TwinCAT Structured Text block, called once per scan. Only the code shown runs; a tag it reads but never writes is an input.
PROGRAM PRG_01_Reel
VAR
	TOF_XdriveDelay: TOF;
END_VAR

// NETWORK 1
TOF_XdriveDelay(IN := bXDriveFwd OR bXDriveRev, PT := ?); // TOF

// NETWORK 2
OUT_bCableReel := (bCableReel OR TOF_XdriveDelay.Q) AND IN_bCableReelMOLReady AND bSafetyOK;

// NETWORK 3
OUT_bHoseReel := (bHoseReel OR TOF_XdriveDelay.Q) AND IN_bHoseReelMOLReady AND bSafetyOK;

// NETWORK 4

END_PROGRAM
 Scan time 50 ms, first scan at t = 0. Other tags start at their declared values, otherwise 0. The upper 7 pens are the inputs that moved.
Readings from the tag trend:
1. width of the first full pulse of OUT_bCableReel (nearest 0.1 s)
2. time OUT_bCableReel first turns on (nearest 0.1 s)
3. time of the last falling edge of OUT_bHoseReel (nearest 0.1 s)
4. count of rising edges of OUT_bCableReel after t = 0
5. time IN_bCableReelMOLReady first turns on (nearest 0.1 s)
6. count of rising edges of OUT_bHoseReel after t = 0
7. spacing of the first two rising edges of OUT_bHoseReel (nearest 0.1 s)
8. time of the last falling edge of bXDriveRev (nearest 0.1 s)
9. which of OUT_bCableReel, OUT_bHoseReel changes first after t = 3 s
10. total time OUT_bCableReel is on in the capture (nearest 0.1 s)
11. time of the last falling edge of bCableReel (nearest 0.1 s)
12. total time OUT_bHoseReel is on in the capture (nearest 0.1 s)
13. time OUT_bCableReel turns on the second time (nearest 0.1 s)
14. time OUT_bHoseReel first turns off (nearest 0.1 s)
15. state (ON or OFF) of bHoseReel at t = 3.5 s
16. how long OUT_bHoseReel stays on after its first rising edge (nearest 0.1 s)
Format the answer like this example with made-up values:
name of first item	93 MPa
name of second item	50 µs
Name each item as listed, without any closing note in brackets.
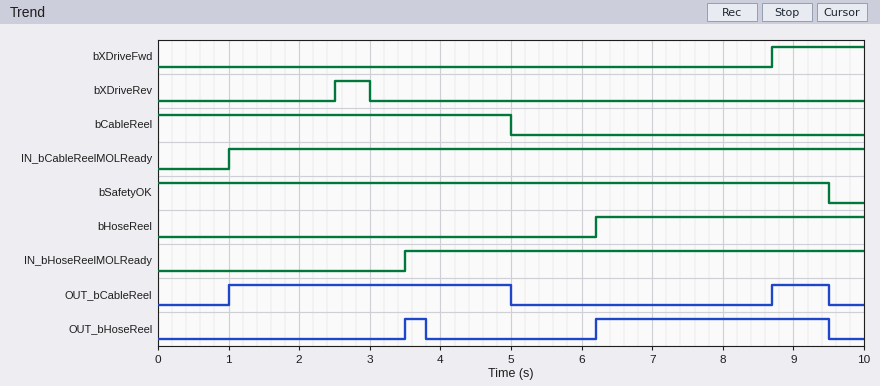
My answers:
width of the first full pulse of OUT_bCableReel	4.0 s
time OUT_bCableReel first turns on	1.0 s
time of the last falling edge of OUT_bHoseReel	9.5 s
count of rising edges of OUT_bCableReel after t = 0	2
time IN_bCableReelMOLReady first turns on	1.0 s
count of rising edges of OUT_bHoseReel after t = 0	2
spacing of the first two rising edges of OUT_bHoseReel	2.7 s
time of the last falling edge of bXDriveRev	3.0 s
which of OUT_bCableReel, OUT_bHoseReel changes first after t = 3 s	OUT_bHoseReel
total time OUT_bCableReel is on in the capture	4.8 s
time of the last falling edge of bCableReel	5.0 s
total time OUT_bHoseReel is on in the capture	3.6 s
time OUT_bCableReel turns on the second time	8.7 s
time OUT_bHoseReel first turns off	3.8 s
state (ON or OFF) of bHoseReel at t = 3.5 s	OFF
how long OUT_bHoseReel stays on after its first rising edge	0.3 s
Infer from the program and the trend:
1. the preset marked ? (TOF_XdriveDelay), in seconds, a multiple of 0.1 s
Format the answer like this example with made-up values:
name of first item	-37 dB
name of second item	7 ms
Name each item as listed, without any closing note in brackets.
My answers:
the preset marked ? (TOF_XdriveDelay), in seconds, a multiple of 0.1 s	0.8 s
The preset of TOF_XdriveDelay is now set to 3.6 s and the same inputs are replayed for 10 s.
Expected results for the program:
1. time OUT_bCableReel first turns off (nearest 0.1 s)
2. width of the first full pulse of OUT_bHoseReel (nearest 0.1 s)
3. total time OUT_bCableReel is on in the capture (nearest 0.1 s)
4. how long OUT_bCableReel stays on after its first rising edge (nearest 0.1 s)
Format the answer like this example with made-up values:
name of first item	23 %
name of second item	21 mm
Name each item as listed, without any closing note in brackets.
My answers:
time OUT_bCableReel first turns off	6.6 s
width of the first full pulse of OUT_bHoseReel	6.0 s
total time OUT_bCableReel is on in the capture	6.4 s
how long OUT_bCableReel stays on after its first rising edge	5.6 s
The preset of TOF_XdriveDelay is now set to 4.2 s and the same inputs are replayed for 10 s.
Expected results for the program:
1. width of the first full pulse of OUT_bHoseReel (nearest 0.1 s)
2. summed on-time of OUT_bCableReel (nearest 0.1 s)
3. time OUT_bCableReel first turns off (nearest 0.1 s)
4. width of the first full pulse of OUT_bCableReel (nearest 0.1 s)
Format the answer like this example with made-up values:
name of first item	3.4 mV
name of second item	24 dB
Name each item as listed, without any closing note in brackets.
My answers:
width of the first full pulse of OUT_bHoseReel	6.0 s
summed on-time of OUT_bCableReel	7.0 s
time OUT_bCableReel first turns off	7.2 s
width of the first full pulse of OUT_bCableReel	6.2 s
